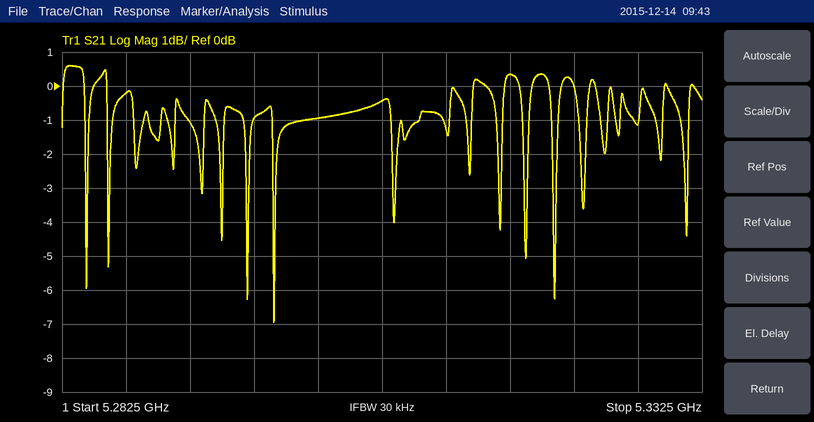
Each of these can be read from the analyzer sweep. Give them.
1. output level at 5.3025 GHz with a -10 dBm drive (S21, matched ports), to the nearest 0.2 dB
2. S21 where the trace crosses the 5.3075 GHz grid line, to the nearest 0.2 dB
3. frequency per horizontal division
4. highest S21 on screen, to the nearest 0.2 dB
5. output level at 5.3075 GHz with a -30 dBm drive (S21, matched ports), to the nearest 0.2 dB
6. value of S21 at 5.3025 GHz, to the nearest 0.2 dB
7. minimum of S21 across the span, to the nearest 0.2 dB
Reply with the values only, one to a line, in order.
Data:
-11.0 dBm
-0.4 dB
5 MHz
0.6 dB
-30.4 dBm
-1.0 dB
-7.0 dB
